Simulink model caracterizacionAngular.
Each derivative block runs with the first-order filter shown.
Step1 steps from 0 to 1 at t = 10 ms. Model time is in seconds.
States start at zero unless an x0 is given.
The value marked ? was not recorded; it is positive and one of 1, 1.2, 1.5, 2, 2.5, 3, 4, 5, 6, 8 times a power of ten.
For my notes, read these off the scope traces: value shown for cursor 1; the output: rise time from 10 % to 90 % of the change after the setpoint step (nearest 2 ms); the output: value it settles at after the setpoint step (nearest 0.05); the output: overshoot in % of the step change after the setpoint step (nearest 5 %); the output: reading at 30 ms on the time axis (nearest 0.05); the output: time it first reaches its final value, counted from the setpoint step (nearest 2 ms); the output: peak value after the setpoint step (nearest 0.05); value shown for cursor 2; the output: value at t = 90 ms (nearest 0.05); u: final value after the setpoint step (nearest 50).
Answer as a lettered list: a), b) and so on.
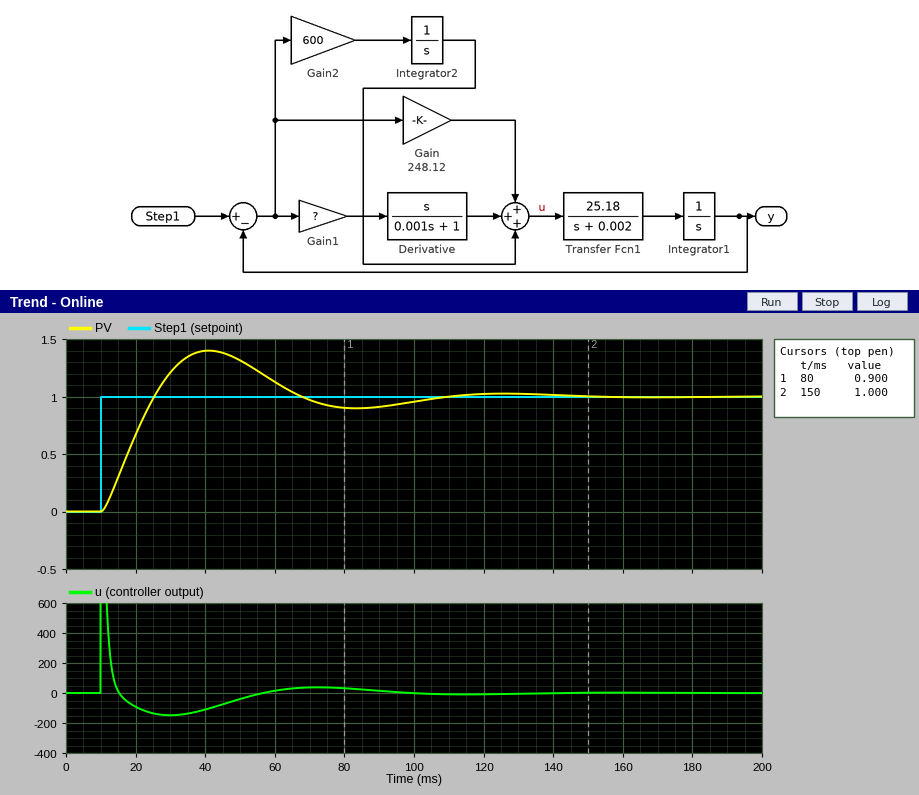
a) 0.900
b) 12 ms
c) 1.00
d) 40 %
e) 1.20
f) 16 ms
g) 1.40
h) 1.000
i) 0.90
j) 0
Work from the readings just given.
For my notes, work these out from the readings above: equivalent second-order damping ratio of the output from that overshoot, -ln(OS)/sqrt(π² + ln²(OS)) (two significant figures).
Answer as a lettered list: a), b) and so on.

a) 0.28
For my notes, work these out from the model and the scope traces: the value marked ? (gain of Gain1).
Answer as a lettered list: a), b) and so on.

a) 2.5
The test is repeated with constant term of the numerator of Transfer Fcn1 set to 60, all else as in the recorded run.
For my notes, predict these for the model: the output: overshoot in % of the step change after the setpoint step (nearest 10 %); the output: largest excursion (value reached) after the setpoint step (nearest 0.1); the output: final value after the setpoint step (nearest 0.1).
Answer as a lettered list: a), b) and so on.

a) 30 %
b) 1.3
c) 1.0
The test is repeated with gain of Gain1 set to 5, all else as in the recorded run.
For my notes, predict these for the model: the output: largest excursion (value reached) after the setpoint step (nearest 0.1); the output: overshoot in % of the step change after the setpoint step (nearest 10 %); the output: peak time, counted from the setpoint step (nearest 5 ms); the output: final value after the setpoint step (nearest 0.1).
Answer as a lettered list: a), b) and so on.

a) 1.2
b) 20 %
c) 25 ms
d) 1.0
